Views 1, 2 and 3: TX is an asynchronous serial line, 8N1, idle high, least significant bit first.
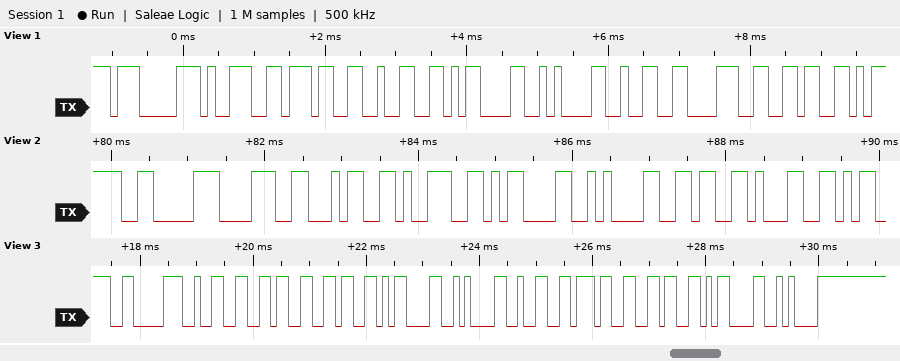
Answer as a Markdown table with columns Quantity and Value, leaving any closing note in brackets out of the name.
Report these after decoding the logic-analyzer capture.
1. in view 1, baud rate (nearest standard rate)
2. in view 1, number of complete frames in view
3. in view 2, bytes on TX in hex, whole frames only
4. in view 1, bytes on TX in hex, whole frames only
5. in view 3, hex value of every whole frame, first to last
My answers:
| Quantity | Value |
|---|---|
| in view 1, baud rate | 9600 baud |
| in view 1, number of complete frames in view | 9 |
| in view 2, bytes on TX in hex, whole frames only | 06 38 34 39 0D 0A 36 31 |
| in view 1, bytes on TX in hex, whole frames only | 07 39 37 32 0D 0A 32 38 36 |
| in view 3, hex value of every whole frame, first to last | 06 32 36 36 0D 0A 32 37 36 0D 0A |
